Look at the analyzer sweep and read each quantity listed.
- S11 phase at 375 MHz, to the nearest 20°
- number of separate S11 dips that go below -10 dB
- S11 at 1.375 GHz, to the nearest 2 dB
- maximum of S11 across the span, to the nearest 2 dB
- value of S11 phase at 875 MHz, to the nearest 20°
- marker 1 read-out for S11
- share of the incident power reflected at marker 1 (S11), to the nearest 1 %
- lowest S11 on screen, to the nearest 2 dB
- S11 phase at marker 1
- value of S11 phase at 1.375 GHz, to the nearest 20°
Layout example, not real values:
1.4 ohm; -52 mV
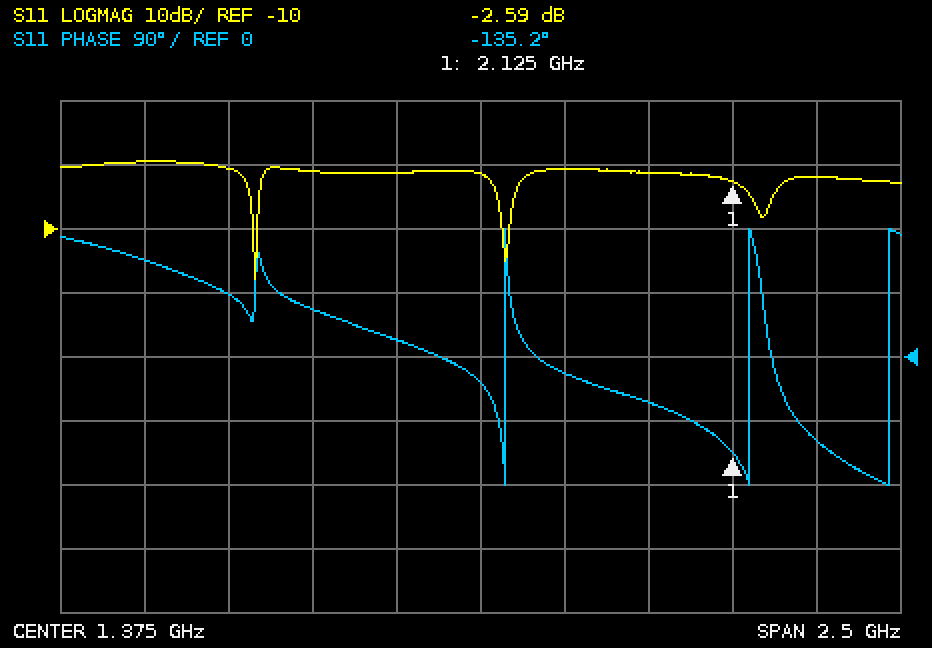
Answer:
140°; 2; -2 dB; 0 dB; 60°; -2.59 dB; 55 %; -18 dB; -135.2°; -40°
